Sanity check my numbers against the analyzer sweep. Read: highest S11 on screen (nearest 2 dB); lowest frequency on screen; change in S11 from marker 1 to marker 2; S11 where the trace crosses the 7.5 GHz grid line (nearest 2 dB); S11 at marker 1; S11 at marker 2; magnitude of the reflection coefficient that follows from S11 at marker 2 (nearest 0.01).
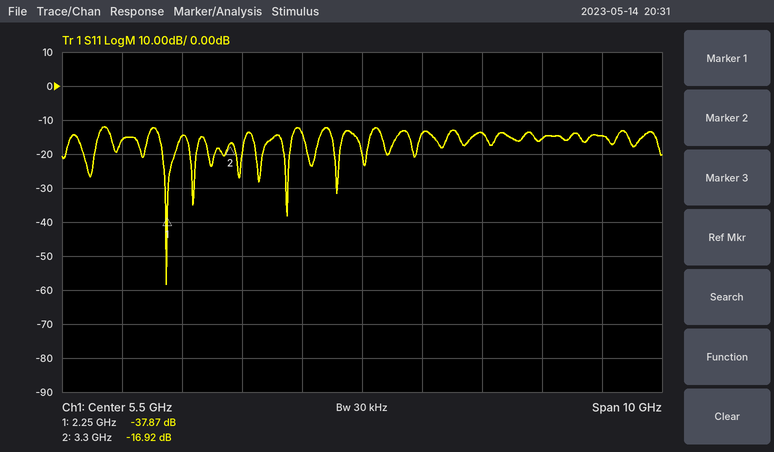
-12 dB
500 MHz
20.95 dB
-14 dB
-37.87 dB
-16.92 dB
0.14
